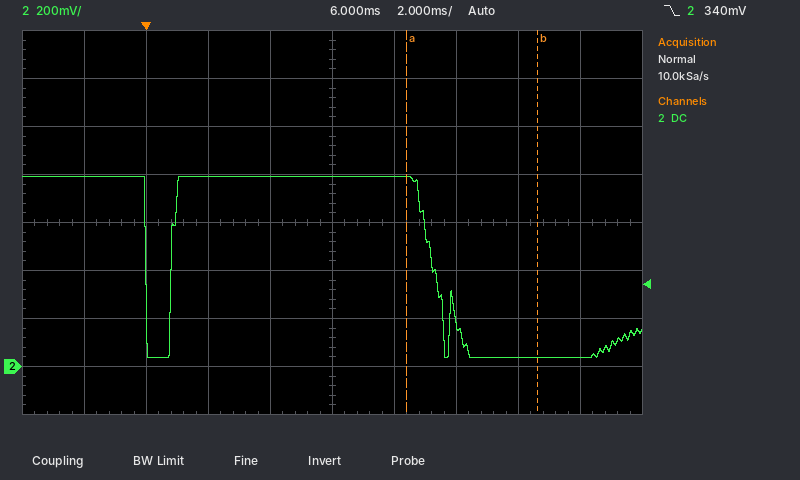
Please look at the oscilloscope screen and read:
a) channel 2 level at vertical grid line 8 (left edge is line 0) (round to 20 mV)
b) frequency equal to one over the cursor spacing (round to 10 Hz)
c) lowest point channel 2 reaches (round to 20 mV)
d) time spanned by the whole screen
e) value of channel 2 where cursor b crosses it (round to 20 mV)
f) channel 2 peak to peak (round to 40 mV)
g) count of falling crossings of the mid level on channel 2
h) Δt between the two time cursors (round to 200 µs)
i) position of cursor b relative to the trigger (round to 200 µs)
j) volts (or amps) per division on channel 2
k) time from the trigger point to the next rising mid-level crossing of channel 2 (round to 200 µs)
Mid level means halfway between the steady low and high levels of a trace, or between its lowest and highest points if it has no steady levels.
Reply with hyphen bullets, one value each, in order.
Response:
- 40 mV
- 240 Hz
- 40 mV
- 20 ms
- 40 mV
- 760 mV
- 2
- 4.2 ms
- +12.6 ms
- 200 mV
- 800 µs
